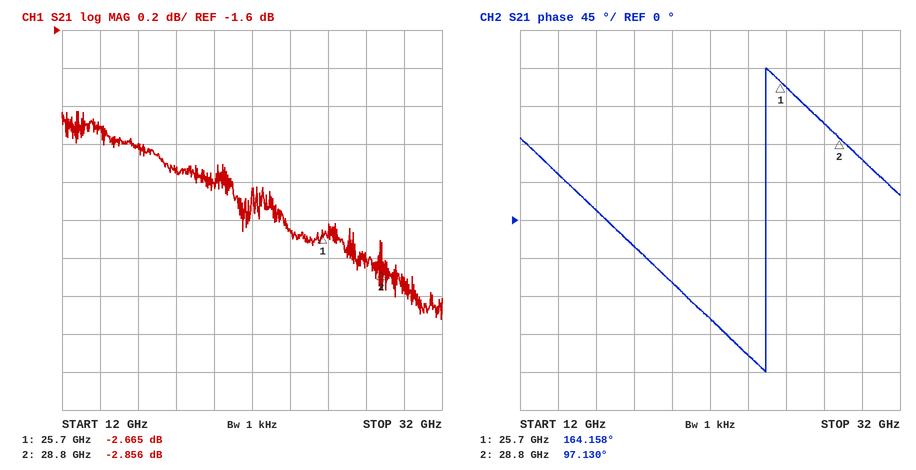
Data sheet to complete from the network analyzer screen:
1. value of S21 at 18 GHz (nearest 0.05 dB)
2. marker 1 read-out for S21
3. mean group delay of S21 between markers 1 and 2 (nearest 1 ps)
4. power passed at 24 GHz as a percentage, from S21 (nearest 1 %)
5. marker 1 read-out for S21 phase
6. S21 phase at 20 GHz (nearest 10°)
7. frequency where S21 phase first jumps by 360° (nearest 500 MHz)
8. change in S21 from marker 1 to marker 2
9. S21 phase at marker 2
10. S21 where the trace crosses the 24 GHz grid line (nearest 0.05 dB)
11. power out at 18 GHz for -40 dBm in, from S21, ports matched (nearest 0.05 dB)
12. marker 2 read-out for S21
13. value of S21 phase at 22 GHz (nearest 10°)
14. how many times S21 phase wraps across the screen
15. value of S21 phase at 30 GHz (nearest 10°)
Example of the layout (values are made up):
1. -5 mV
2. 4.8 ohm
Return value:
1. -2.35 dB
2. -2.665 dB
3. 60 ps
4. 54 %
5. 164.158°
6. -70°
7. 25.0 GHz
8. -0.191 dB
9. 97.130°
10. -2.65 dB
11. -42.35 dBm
12. -2.856 dB
13. -120°
14. 1
15. 70°
